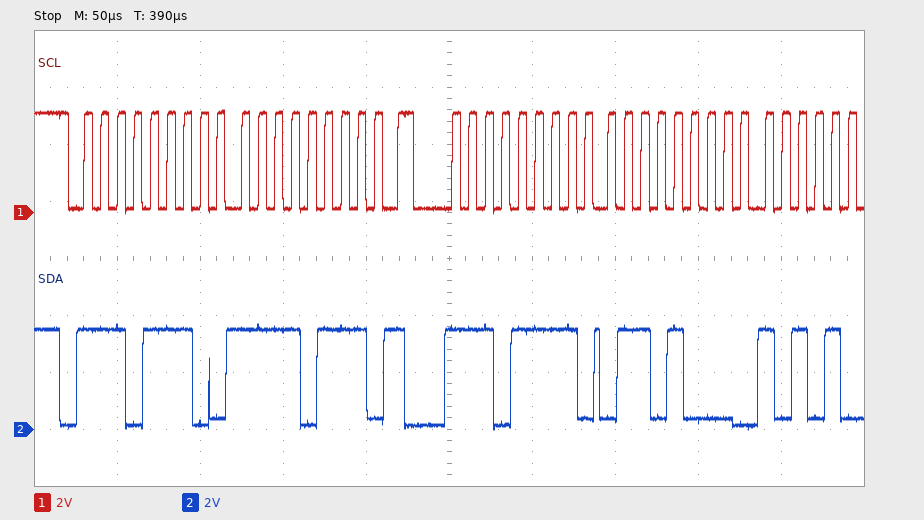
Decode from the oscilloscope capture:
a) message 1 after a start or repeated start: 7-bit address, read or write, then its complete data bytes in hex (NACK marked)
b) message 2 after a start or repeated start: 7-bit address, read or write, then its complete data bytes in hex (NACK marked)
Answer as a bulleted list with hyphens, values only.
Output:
- 0x77 write: F7
- 0x77 read: 68
